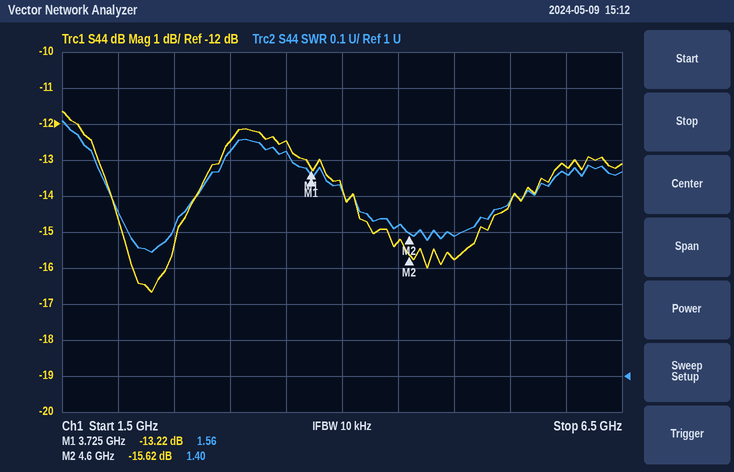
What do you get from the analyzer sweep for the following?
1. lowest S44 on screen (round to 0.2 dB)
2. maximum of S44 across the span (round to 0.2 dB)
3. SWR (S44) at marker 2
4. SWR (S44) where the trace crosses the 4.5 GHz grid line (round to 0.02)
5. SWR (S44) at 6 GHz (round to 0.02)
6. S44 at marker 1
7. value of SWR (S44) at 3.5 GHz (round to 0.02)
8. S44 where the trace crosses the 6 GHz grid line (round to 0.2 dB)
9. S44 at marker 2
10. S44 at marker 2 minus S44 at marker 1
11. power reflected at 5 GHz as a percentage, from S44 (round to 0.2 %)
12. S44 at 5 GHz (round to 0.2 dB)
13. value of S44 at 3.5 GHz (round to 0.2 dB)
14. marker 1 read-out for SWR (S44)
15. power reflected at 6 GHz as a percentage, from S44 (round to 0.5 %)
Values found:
-16.6 dB
-11.6 dB
1.40
1.42
1.56
-13.22 dB
1.62
-13.2 dB
-15.62 dB
-2.40 dB
2.6 %
-15.8 dB
-12.4 dB
1.56
5.0 %
